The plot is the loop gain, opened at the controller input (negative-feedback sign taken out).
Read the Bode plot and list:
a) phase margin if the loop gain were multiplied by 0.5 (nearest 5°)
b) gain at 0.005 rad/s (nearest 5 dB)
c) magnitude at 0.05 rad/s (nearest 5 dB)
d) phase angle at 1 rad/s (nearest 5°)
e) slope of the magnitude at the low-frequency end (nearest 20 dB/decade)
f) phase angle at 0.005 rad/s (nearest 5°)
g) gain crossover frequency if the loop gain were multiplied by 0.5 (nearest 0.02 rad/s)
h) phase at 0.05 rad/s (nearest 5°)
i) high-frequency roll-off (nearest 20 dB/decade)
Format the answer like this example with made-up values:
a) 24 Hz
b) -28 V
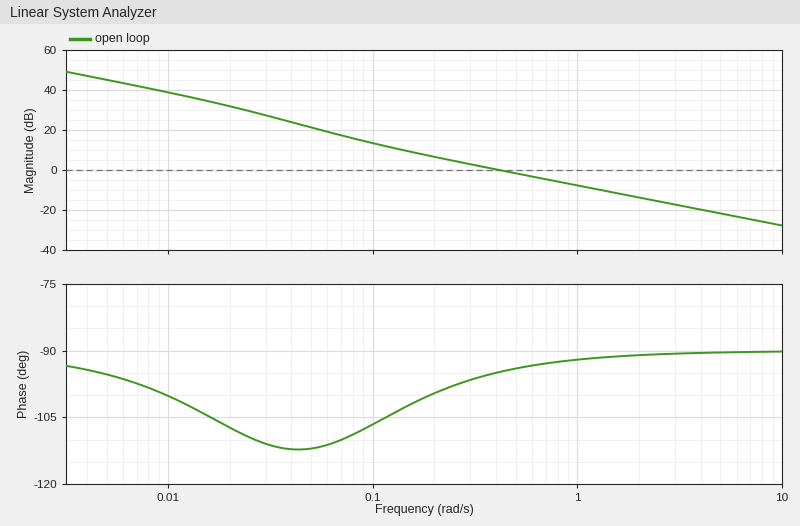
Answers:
a) 80°
b) 45 dB
c) 20 dB
d) -90°
e) -20 dB/decade
f) -95°
g) 0.22 rad/s
h) -110°
i) -20 dB/decade
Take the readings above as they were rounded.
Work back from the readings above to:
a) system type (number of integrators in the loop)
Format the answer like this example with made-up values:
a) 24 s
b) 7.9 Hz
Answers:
a) 1
